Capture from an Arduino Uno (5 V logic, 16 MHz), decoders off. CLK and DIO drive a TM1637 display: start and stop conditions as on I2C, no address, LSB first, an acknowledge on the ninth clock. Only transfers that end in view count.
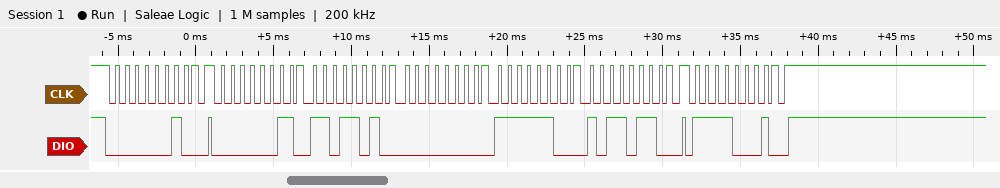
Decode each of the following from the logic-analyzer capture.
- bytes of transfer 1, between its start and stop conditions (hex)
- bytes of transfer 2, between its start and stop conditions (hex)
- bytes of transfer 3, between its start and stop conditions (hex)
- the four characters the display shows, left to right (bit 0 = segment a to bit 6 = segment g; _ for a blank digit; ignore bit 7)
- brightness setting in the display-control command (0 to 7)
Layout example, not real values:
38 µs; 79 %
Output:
40; C0 5B 00 3F 6D; 8F; 2_05; 7
